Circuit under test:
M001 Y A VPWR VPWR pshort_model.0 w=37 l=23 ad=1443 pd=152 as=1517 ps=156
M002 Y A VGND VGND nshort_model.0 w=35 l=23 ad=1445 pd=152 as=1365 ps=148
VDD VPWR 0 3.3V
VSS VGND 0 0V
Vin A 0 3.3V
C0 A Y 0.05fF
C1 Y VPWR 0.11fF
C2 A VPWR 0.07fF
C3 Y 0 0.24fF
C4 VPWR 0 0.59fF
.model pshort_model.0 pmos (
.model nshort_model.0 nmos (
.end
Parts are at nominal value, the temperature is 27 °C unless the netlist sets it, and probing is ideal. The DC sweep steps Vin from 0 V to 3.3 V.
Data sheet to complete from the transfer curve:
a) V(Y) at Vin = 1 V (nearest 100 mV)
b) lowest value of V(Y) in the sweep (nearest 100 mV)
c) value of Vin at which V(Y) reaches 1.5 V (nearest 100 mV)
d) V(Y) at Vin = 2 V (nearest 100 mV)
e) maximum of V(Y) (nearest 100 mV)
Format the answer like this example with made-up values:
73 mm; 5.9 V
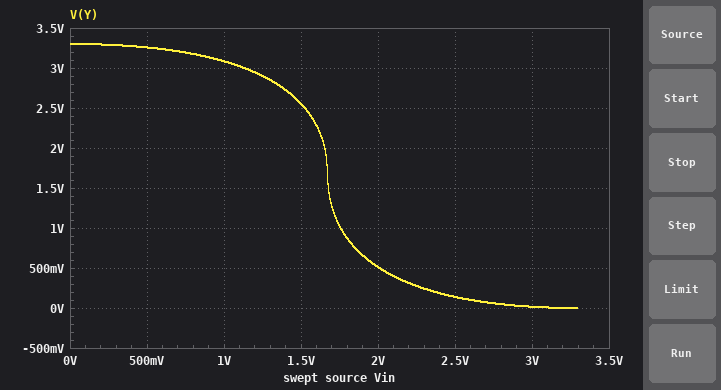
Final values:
3.1 V; 0 V; 1.7 V; 500 mV; 3.3 V
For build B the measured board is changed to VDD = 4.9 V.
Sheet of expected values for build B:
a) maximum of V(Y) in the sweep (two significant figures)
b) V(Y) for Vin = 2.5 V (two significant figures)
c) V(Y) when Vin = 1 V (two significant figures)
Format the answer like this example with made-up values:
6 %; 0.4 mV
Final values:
4.9 V; 2.1 V; 4.8 V
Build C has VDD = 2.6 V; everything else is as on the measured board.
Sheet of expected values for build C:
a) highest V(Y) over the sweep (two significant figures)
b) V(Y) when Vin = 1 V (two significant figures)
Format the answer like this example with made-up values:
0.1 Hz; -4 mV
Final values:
2.6 V; 2.3 V
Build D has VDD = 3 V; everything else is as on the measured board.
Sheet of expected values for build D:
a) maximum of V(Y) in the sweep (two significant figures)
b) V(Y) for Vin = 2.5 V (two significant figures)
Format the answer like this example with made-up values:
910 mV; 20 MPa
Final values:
3.0 V; 53 mV
